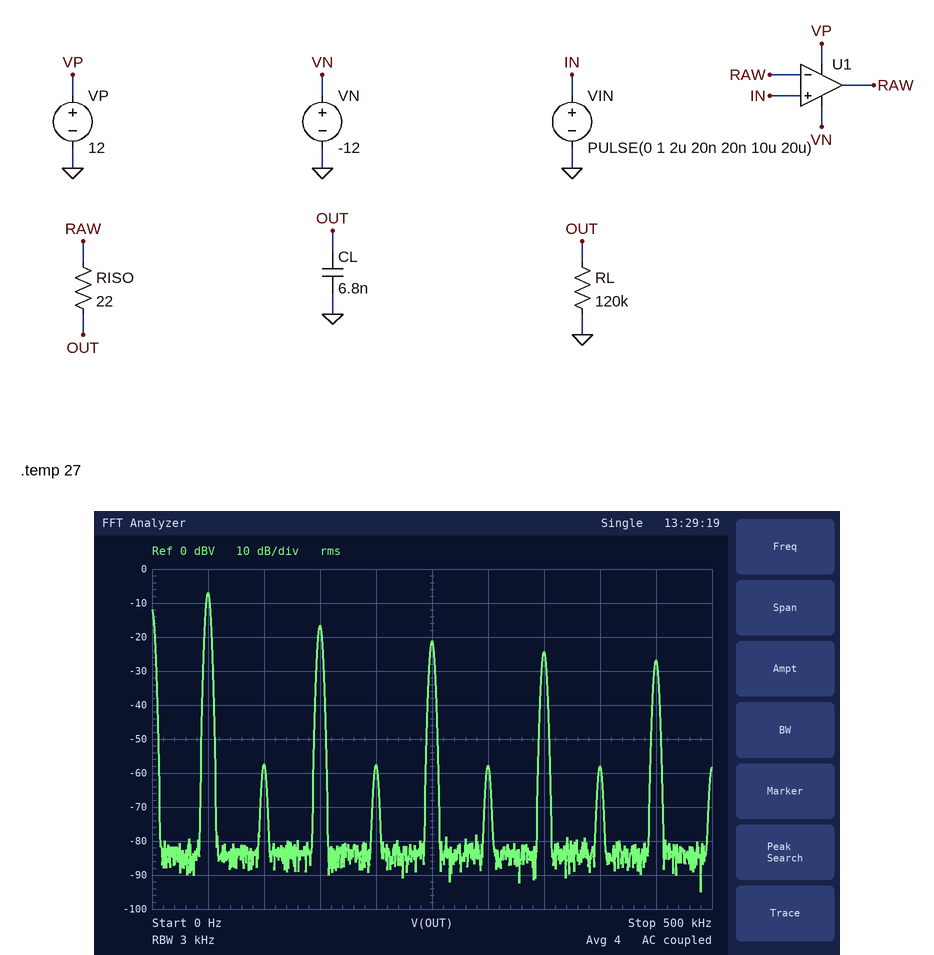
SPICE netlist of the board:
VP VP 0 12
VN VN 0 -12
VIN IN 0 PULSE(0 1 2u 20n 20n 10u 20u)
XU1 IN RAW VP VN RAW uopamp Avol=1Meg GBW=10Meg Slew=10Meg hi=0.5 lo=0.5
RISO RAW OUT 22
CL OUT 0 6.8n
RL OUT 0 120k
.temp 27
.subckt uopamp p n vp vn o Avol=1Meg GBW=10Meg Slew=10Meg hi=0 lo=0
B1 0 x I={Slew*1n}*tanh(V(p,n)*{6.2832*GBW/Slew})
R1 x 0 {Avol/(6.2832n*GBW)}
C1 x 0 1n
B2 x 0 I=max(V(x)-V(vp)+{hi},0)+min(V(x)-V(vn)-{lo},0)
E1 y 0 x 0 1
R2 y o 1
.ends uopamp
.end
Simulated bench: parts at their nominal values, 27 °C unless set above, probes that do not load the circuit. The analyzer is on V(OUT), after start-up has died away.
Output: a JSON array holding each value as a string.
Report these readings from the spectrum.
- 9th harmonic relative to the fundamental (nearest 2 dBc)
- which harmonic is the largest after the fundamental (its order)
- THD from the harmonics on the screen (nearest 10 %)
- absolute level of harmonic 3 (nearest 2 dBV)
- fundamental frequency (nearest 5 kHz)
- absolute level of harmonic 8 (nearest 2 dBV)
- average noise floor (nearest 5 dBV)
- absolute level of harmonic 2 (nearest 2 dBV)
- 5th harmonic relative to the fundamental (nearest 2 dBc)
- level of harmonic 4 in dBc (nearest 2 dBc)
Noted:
["-20 dBc", "3", "40 %", "-16 dBV", "50 kHz", "-58 dBV", "-85 dBV", "-58 dBV", "-14 dBc", "-50 dBc"]
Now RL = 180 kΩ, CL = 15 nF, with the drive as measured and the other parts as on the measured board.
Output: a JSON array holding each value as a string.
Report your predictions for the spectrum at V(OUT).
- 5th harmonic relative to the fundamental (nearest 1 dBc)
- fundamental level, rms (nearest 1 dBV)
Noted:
["-15 dBc", "-7 dBV"]
